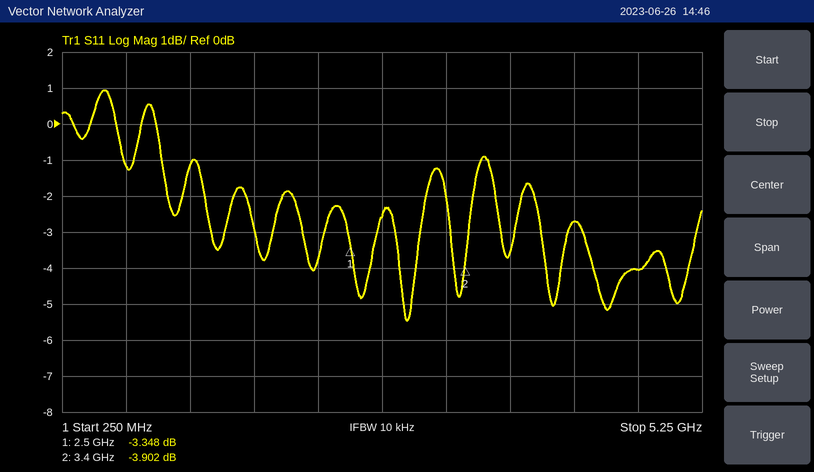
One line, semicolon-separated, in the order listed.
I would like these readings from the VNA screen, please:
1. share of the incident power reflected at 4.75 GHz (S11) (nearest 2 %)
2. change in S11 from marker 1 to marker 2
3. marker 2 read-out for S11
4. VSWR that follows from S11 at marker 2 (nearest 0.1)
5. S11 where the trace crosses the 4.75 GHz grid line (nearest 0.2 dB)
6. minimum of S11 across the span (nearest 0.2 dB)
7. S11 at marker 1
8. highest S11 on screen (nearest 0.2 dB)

40 %; -0.554 dB; -3.902 dB; 4.5; -4.0 dB; -5.4 dB; -3.348 dB; 1.0 dB
